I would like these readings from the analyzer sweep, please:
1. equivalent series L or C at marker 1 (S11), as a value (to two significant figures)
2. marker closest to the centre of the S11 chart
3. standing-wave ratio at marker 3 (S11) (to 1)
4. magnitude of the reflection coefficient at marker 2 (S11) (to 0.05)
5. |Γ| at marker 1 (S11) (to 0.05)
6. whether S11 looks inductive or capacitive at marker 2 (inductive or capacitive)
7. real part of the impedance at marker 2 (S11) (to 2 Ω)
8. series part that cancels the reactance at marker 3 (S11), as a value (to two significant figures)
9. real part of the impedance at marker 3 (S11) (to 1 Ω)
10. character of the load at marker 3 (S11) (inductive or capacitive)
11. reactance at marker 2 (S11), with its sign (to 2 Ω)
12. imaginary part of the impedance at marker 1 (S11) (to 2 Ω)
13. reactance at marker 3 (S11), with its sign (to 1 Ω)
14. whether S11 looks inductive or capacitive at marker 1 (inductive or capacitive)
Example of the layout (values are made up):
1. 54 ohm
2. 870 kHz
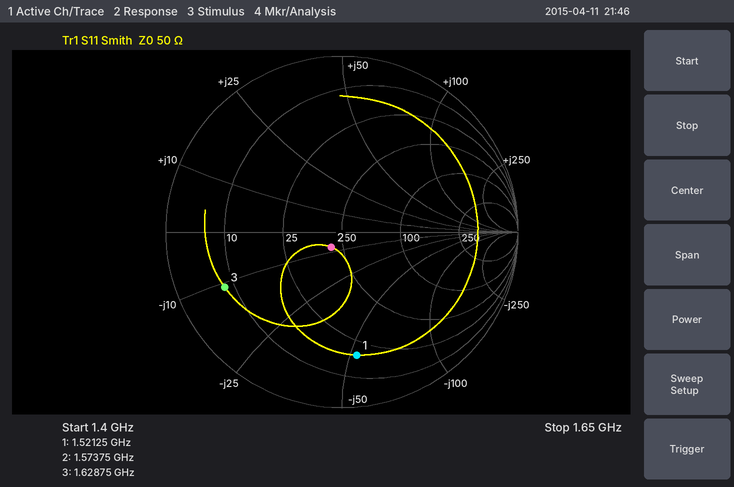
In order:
1. 2.0 pF
2. marker 2
3. 7
4. 0.10
5. 0.70
6. capacitive
7. 44 Ω
8. 1.1 nH
9. 8 Ω
10. capacitive
11. -8 Ω
12. -52 Ω
13. -11 Ω
14. capacitive
